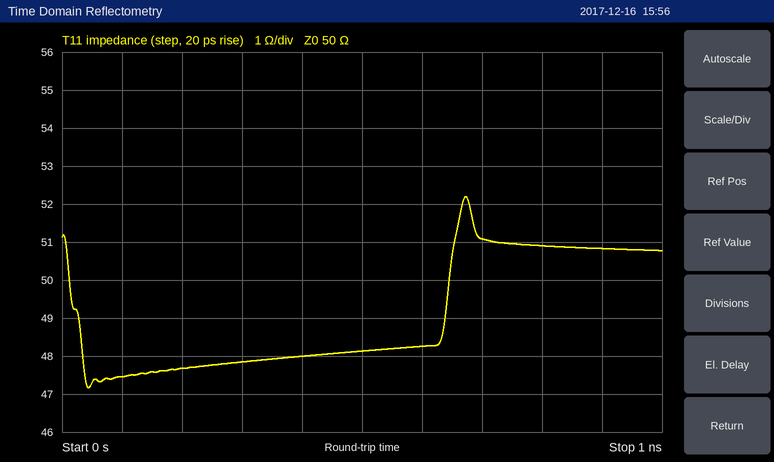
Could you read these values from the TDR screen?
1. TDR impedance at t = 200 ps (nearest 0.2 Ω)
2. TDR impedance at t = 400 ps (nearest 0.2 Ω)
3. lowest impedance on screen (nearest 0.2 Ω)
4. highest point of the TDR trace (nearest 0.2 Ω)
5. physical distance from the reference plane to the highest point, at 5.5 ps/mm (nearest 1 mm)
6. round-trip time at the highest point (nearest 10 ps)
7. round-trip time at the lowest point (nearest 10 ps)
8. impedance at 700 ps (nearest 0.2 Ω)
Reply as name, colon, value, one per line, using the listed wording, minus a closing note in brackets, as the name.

TDR impedance at t = 200 ps: 47.6 Ω
TDR impedance at t = 400 ps: 48.0 Ω
lowest impedance on screen: 47.2 Ω
highest point of the TDR trace: 52.2 Ω
physical distance from the reference plane to the highest point, at 5.5 ps/mm: 61 mm
round-trip time at the highest point: 670 ps
round-trip time at the lowest point: 40 ps
impedance at 700 ps: 51.0 Ω
